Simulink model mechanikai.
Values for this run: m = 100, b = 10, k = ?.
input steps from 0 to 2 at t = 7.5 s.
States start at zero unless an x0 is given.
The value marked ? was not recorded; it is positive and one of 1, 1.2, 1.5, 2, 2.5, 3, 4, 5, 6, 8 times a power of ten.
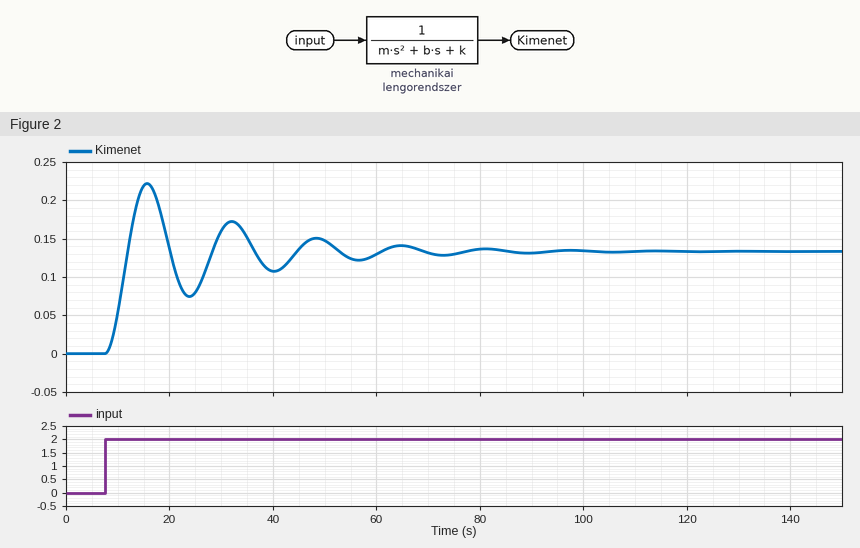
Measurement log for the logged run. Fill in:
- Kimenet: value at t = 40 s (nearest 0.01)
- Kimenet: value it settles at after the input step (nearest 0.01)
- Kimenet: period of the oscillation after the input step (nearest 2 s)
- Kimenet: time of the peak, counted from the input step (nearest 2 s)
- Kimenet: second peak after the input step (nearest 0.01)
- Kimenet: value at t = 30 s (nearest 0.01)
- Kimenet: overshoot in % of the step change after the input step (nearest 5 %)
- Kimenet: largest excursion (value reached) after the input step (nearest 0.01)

0.11
0.13
16 s
8 s
0.17
0.16
65 %
0.22
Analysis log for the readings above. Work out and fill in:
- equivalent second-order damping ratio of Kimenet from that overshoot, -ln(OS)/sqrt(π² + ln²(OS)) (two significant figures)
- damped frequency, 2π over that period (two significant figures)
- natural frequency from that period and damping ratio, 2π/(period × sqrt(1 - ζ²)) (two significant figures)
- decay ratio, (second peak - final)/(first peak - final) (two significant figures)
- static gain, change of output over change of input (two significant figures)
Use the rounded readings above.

0.14
0.39 rad/s
0.40 rad/s
0.44
0.065
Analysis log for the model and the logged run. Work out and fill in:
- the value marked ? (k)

15
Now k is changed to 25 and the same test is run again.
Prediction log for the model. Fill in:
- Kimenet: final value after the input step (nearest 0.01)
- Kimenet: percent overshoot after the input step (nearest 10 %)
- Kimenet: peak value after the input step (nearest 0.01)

0.08
70 %
0.14
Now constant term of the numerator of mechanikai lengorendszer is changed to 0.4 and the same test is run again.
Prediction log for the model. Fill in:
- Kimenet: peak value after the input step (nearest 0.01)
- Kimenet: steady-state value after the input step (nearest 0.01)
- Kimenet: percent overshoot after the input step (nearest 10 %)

0.09
0.05
70 %
